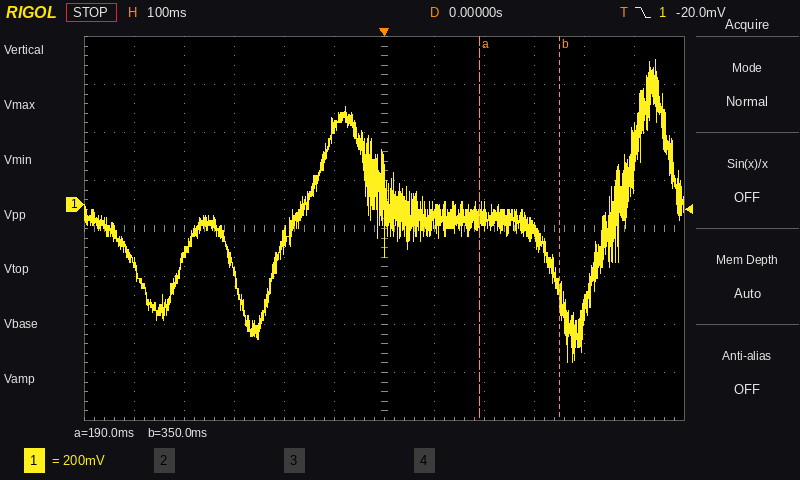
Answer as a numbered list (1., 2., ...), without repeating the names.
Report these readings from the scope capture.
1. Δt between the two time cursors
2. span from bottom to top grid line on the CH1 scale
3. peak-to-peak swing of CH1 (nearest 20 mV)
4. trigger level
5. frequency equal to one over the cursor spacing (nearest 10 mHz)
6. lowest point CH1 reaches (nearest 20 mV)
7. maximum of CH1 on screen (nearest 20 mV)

1. 160 ms
2. 1.6 V
3. 1.26 V
4. -20.0 mV
5. 6.25 Hz
6. -660 mV
7. 600 mV
